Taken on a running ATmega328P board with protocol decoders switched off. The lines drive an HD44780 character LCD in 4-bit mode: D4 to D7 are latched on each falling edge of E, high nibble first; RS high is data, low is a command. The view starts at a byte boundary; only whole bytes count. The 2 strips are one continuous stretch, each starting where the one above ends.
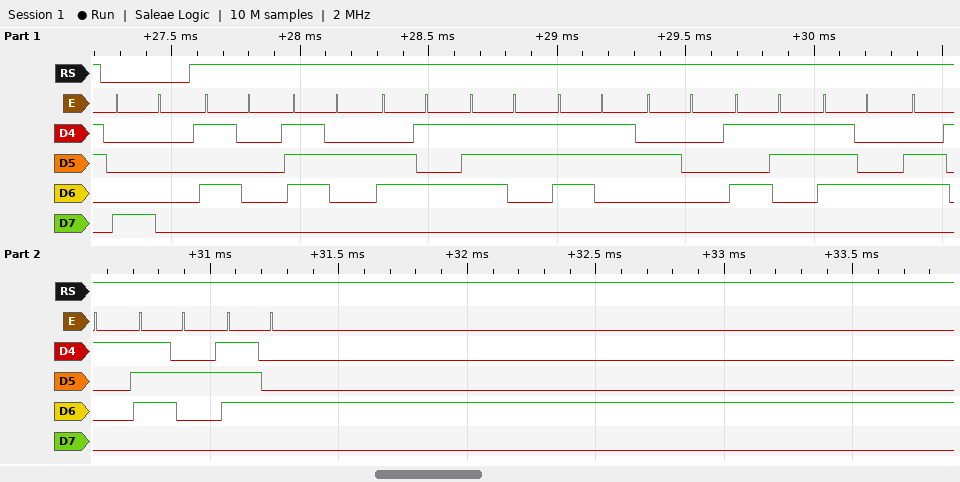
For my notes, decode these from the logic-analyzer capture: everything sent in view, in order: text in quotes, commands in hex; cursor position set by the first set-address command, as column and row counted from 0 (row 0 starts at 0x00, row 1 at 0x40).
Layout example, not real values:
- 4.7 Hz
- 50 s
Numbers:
- 0x80 "Press Start"
- column 0, row 0
